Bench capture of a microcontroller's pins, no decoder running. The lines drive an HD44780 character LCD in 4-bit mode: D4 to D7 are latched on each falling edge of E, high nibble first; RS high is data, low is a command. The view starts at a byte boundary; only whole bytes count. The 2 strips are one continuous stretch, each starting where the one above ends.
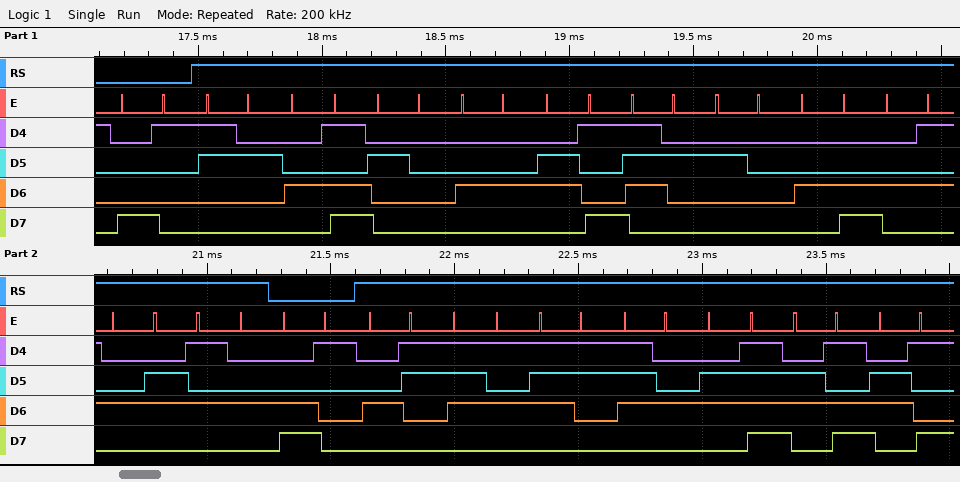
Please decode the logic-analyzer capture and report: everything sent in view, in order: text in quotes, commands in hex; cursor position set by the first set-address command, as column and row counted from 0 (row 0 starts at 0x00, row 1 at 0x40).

0x81 "2M Dir LEFT" 0xC1 "Customi"
column 1, row 0
